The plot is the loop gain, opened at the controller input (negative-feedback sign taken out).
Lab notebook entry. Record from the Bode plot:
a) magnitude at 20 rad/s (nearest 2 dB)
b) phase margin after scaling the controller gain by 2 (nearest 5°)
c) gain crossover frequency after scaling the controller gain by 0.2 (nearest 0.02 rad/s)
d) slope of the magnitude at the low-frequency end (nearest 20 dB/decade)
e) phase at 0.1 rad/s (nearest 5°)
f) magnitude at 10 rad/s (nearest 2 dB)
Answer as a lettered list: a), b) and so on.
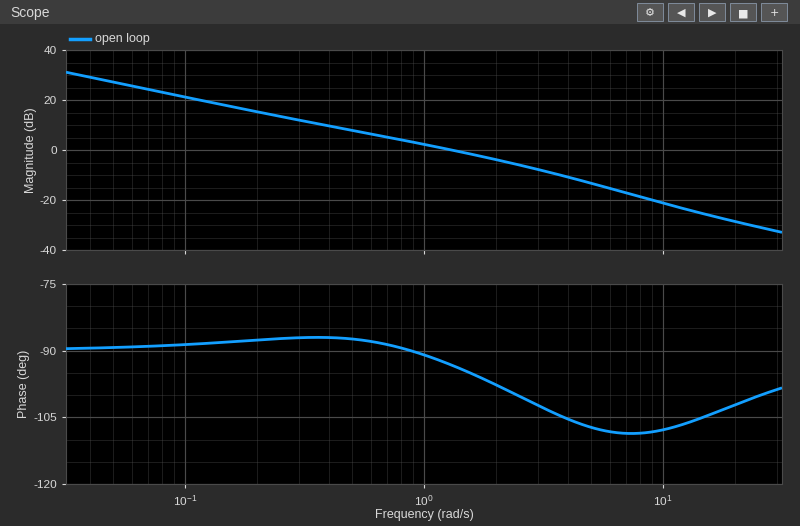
a) -28 dB
b) 80°
c) 0.24 rad/s
d) -20 dB/decade
e) -90°
f) -22 dB
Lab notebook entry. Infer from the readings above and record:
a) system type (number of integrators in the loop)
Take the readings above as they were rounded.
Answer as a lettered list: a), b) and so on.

a) 1
